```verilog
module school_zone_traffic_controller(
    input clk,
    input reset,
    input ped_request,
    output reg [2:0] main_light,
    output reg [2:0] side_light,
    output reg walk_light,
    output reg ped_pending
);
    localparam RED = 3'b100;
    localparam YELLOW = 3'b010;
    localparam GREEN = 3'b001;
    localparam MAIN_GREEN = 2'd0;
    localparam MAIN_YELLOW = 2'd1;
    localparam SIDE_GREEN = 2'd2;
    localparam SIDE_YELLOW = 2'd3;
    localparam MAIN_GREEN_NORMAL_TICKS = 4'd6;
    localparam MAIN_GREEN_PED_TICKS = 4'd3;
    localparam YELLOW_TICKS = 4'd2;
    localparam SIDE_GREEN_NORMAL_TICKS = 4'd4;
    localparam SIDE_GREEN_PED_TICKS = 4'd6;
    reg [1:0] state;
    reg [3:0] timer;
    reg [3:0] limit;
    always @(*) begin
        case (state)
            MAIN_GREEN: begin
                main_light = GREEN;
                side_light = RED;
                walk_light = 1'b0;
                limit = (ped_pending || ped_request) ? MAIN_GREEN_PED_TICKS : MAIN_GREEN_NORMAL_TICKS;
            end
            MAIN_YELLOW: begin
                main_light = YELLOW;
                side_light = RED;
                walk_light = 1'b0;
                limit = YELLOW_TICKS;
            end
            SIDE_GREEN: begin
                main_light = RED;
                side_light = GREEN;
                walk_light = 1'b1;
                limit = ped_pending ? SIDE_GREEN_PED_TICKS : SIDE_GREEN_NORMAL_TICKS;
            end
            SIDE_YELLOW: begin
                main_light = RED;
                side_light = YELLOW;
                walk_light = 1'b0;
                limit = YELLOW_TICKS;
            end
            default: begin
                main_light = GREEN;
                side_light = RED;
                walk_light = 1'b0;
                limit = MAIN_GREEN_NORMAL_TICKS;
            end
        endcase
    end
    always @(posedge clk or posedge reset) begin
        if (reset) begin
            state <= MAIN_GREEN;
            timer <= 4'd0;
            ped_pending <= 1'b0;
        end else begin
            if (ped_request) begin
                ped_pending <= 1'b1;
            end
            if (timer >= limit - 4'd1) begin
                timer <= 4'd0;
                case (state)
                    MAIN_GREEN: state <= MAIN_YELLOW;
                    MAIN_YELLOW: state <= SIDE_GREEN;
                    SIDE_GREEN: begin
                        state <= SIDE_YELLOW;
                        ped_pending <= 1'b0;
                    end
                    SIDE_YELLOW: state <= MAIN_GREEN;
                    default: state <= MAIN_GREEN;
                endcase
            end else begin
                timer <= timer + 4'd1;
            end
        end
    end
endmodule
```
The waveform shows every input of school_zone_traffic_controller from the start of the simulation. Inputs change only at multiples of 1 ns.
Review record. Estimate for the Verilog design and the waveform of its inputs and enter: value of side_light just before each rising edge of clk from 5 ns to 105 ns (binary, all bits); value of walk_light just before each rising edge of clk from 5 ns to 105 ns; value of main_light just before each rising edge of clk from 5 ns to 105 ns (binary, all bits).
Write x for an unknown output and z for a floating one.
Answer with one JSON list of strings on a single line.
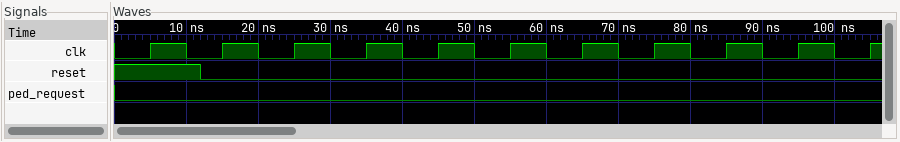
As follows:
["100, 100, 100, 100, 100, 100, 100, 100, 100, 001, 001", "0 0 0 0 0 0 0 0 0 1 1", "001, 001, 001, 001, 001, 001, 001, 010, 010, 100, 100"]
